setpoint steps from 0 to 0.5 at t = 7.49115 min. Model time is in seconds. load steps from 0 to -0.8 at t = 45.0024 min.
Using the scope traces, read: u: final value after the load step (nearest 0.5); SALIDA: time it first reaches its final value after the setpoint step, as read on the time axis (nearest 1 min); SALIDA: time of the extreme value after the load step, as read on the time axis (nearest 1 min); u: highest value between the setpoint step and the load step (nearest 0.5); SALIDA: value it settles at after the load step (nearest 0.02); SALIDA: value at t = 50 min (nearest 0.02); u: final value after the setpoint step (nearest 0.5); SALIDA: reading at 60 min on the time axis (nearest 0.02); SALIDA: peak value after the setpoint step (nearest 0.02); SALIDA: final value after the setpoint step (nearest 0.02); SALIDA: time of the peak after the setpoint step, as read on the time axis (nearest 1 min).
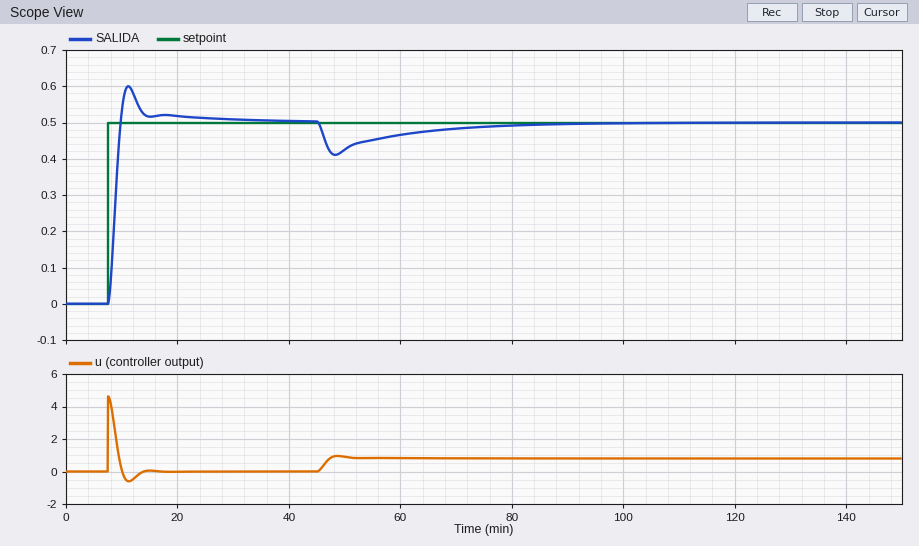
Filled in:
1.0
10 min
48 min
4.5
0.50
0.42
0.0
0.46
0.60
0.50
11 min
